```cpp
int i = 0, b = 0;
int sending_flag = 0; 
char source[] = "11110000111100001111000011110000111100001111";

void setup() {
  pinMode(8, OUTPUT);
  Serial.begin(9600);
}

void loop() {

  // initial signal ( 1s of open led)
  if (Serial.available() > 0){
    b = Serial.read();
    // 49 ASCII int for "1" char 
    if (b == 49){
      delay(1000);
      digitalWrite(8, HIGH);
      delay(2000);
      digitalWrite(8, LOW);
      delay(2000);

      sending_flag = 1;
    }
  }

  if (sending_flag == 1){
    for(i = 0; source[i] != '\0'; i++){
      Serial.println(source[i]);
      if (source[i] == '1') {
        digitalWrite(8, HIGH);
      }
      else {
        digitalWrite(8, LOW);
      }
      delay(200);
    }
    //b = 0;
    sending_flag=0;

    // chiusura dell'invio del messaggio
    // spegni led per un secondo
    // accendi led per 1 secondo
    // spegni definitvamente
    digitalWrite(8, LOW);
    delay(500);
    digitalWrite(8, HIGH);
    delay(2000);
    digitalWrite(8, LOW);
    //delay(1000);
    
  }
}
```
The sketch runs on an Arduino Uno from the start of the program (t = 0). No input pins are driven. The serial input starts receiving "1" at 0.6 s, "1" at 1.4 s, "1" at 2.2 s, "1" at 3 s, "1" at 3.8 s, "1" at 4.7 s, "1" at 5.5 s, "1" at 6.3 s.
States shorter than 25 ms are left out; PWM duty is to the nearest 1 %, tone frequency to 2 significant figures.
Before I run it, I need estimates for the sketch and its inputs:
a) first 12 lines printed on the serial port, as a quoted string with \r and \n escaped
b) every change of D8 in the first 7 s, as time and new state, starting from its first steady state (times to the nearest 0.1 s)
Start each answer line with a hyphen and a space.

- "1\r\n1\r\n1\r\n1\r\n0\r\n0\r\n0\r\n0\r\n1\r\n1\r\n1\r\n1\r\n"
- 0 s low; 1.6 s high; 3.6 s low; 5.6 s high; 6.4 s low
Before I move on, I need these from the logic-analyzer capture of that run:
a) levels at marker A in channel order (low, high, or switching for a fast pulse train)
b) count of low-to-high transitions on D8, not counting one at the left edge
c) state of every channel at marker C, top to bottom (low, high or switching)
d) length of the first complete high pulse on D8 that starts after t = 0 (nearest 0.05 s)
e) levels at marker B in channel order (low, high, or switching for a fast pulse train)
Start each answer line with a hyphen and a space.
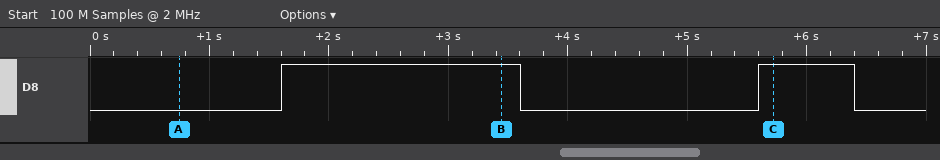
- D8 low
- 2
- D8 high
- 2.00 s
- D8 high
